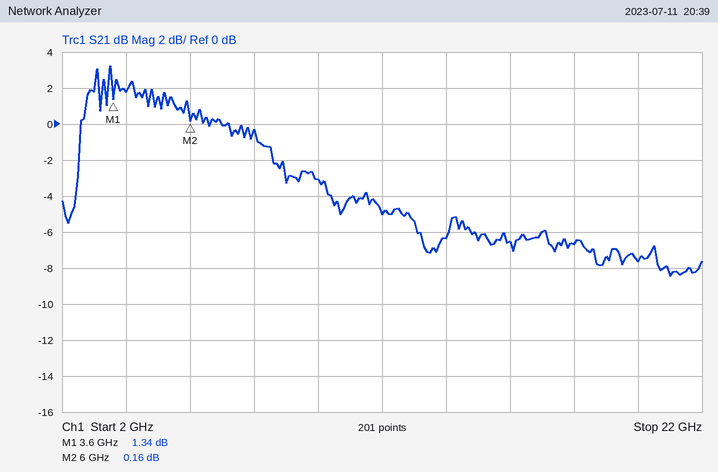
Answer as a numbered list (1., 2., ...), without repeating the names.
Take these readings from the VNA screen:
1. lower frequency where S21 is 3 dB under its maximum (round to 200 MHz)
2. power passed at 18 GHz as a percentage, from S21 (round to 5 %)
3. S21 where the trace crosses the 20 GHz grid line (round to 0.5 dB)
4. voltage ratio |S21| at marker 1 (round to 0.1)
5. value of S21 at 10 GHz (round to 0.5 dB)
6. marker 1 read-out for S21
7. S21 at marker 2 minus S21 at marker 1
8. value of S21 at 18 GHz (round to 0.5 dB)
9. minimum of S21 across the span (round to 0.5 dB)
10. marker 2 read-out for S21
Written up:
1. 2.6 GHz
2. 20 %
3. -7.5 dB
4. 1.2
5. -3.0 dB
6. 1.34 dB
7. -1.18 dB
8. -6.5 dB
9. -8.5 dB
10. 0.16 dB
